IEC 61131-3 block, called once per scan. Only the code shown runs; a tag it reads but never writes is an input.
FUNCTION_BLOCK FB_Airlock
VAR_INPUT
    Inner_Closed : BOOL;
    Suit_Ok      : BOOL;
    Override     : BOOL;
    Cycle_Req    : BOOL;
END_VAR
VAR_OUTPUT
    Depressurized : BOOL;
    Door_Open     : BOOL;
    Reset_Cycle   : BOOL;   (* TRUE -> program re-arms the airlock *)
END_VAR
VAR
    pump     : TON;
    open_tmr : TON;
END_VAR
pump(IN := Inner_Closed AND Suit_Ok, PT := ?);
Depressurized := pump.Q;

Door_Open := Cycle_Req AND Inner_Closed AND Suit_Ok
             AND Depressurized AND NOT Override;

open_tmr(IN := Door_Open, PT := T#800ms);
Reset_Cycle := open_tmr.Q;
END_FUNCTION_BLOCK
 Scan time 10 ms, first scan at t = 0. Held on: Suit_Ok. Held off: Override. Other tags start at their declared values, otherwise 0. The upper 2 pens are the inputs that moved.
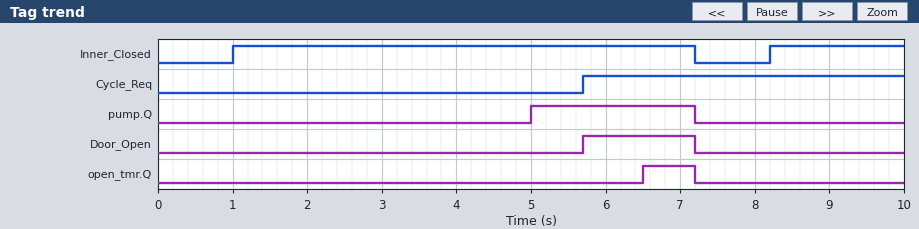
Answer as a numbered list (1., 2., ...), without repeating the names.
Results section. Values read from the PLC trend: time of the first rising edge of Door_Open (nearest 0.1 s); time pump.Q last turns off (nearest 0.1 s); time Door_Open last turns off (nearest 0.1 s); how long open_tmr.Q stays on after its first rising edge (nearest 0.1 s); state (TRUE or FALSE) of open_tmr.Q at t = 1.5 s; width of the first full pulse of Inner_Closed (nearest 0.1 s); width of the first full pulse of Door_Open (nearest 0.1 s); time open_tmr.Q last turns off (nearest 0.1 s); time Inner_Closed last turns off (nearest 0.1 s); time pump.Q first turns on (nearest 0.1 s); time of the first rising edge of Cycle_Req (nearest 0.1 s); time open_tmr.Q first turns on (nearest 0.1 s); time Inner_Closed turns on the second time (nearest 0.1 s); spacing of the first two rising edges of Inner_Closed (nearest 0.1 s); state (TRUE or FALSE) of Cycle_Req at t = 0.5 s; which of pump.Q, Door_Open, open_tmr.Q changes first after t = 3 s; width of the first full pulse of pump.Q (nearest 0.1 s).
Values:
1. 5.7 s
2. 7.2 s
3. 7.2 s
4. 0.7 s
5. FALSE
6. 6.2 s
7. 1.5 s
8. 7.2 s
9. 7.2 s
10. 5.0 s
11. 5.7 s
12. 6.5 s
13. 8.2 s
14. 7.2 s
15. FALSE
16. pump.Q
17. 2.2 s
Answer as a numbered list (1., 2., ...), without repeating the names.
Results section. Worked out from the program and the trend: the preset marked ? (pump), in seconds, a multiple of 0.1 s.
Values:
1. 4.0 s
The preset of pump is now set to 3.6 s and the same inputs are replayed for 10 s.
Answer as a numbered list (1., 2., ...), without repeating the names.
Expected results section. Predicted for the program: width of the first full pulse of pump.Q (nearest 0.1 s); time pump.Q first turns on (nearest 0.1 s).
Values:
1. 2.6 s
2. 4.6 s
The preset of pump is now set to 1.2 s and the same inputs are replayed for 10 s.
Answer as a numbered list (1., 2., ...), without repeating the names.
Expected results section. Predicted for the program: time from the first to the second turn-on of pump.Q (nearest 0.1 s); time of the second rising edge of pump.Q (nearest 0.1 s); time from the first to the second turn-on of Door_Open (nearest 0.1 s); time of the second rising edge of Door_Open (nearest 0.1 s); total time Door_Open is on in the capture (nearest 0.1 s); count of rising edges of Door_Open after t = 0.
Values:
1. 7.2 s
2. 9.4 s
3. 3.7 s
4. 9.4 s
5. 2.1 s
6. 2
